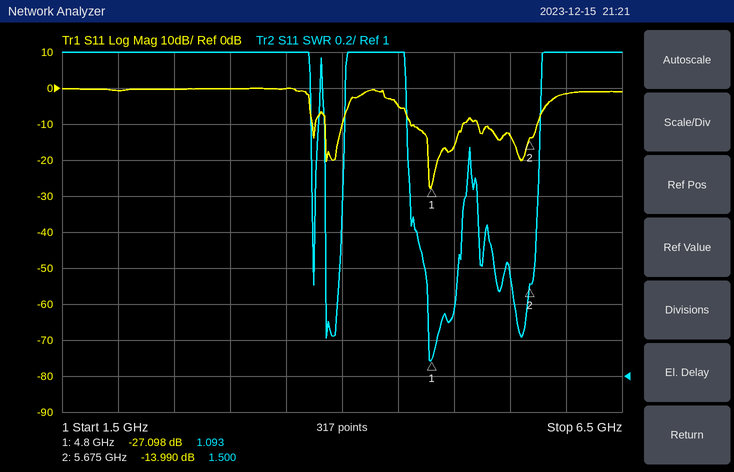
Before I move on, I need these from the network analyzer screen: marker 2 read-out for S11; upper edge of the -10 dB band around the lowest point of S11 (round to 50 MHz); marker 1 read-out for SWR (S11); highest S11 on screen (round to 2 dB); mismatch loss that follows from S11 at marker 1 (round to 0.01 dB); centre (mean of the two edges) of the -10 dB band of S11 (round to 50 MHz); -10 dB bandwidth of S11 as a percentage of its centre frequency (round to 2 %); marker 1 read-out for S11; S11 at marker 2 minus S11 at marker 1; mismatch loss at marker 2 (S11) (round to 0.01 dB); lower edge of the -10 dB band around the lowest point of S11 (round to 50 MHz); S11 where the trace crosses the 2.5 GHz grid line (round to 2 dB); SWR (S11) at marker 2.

-13.990 dB
5.10 GHz
1.093
0 dB
0.01 dB
4.85 GHz
10 %
-27.098 dB
13.108 dB
0.18 dB
4.60 GHz
0 dB
1.500
